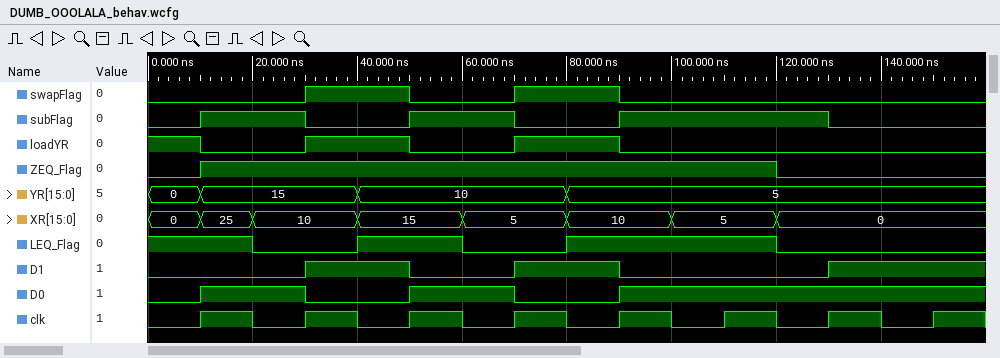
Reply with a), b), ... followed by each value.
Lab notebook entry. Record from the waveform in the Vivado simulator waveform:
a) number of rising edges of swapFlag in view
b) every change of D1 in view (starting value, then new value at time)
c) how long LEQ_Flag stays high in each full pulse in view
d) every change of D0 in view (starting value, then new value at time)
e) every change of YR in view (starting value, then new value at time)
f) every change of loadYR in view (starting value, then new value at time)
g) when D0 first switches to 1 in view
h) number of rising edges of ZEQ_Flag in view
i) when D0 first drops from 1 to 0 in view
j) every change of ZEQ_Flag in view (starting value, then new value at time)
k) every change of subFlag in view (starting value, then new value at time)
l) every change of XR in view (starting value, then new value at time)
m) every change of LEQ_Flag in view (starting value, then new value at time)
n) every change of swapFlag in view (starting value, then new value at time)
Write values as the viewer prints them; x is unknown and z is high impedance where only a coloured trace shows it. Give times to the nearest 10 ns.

a) 2
b) 0, 1 at 30 ns, 0 at 50 ns, 1 at 70 ns, 0 at 90 ns, 1 at 130 ns
c) 20 ns, 40 ns
d) 0, 1 at 10 ns, 0 at 30 ns, 1 at 50 ns, 0 at 70 ns, 1 at 90 ns
e) 0, 15 at 10 ns, 10 at 40 ns, 5 at 80 ns
f) 1, 0 at 10 ns, 1 at 30 ns, 0 at 50 ns, 1 at 70 ns, 0 at 90 ns
g) 10 ns
h) 1
i) 30 ns
j) 0, 1 at 10 ns, 0 at 120 ns
k) 0, 1 at 10 ns, 0 at 30 ns, 1 at 50 ns, 0 at 70 ns, 1 at 90 ns, 0 at 130 ns
l) 0, 25 at 10 ns, 10 at 20 ns, 15 at 40 ns, 5 at 60 ns, 10 at 80 ns, 5 at 100 ns, 0 at 120 ns
m) 1, 0 at 20 ns, 1 at 40 ns, 0 at 60 ns, 1 at 80 ns, 0 at 120 ns
n) 0, 1 at 30 ns, 0 at 50 ns, 1 at 70 ns, 0 at 90 ns
